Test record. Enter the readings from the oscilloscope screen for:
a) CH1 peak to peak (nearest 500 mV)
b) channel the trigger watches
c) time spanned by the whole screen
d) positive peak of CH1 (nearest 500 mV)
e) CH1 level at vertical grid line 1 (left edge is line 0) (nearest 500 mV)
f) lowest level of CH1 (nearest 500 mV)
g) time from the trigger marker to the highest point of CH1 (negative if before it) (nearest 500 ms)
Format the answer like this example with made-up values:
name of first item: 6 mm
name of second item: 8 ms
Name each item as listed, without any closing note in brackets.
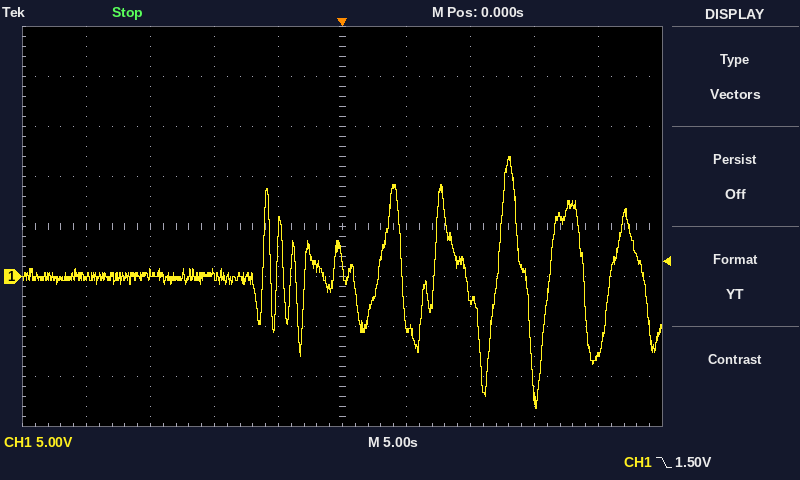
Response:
CH1 peak to peak: 25.0 V
channel the trigger watches: CH1
time spanned by the whole screen: 50 s
positive peak of CH1: 12.0 V
CH1 level at vertical grid line 1 (left edge is line 0): 0.0 V
lowest level of CH1: -13.0 V
time from the trigger marker to the highest point of CH1 (negative if before it): +13.0 s
